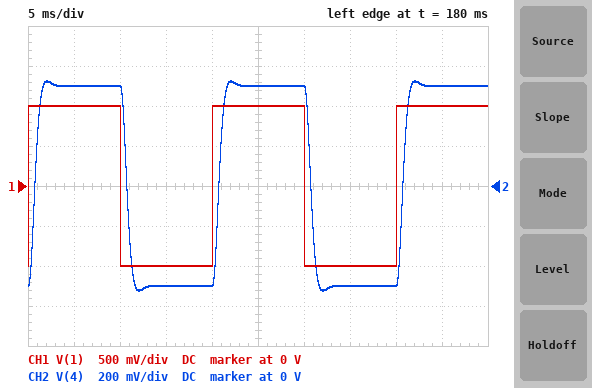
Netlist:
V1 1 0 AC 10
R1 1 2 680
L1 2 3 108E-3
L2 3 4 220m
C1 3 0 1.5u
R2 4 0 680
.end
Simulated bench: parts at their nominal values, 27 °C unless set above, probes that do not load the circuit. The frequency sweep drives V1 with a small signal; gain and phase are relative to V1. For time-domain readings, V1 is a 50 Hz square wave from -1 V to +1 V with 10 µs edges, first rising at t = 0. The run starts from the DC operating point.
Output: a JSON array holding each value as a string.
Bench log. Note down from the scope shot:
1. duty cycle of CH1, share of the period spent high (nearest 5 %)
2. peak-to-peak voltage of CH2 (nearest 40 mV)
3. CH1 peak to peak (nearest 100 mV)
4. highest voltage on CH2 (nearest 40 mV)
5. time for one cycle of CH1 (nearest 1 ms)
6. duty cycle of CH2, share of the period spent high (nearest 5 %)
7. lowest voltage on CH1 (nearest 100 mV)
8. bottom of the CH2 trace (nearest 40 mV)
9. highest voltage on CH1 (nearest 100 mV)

["50 %", "1.04 V", "2.0 V", "520 mV", "20 ms", "50 %", "-1.0 V", "-520 mV", "1.0 V"]
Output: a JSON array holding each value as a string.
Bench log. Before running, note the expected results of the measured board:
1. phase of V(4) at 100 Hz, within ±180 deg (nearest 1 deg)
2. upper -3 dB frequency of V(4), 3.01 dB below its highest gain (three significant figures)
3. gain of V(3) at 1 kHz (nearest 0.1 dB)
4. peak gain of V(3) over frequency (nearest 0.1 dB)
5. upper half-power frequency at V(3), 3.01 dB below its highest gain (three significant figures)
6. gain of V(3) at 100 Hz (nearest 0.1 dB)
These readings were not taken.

["-27 deg", "358 Hz", "-17.9 dB", "-6.0 dB", "476 Hz", "-6.0 dB"]
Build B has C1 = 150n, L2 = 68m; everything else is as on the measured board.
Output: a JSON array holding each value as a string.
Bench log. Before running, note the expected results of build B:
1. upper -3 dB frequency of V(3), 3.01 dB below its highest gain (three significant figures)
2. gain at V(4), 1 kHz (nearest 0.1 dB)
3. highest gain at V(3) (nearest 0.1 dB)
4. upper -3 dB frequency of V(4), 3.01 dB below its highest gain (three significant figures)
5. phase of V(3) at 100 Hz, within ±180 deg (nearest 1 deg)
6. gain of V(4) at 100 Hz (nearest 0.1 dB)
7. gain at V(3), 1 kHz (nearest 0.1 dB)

["2.33 kHz", "-6.4 dB", "-3.3 dB", "2.11 kHz", "-3 deg", "-6.0 dB", "-5.0 dB"]
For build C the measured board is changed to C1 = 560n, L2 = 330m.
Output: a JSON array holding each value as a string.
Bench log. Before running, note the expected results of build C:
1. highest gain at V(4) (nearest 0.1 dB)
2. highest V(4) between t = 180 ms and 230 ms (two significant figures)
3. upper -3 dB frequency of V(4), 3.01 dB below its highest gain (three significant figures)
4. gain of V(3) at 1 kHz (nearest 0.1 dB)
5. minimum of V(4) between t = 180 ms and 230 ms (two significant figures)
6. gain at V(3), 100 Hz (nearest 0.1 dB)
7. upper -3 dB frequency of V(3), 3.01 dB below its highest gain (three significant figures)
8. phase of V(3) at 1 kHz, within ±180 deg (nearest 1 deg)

["-6.0 dB", "560 mV", "618 Hz", "-7.6 dB", "-560 mV", "-5.7 dB", "844 Hz", "-114 deg"]
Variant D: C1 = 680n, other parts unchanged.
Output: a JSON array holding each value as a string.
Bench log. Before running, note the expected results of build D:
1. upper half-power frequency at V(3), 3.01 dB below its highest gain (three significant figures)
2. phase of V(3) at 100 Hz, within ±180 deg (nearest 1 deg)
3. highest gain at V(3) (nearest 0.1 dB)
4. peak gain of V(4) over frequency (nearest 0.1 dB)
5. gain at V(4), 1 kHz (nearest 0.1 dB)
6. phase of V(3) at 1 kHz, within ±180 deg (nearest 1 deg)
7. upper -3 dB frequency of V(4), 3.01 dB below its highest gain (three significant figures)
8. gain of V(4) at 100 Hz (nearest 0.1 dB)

["831 Hz", "-6 deg", "-3.9 dB", "-6.0 dB", "-16.7 dB", "-116 deg", "651 Hz", "-6.0 dB"]
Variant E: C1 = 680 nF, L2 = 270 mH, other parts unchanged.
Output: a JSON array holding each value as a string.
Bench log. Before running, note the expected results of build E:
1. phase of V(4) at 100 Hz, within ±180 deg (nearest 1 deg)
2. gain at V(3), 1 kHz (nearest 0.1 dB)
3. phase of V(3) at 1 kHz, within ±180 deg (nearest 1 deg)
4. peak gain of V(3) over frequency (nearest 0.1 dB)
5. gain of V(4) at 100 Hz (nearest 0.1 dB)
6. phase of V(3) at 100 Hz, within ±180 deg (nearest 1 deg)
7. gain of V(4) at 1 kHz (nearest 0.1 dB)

["-18 deg", "-9.7 dB", "-118 deg", "-3.4 dB", "-6.0 dB", "-4 deg", "-18.3 dB"]
